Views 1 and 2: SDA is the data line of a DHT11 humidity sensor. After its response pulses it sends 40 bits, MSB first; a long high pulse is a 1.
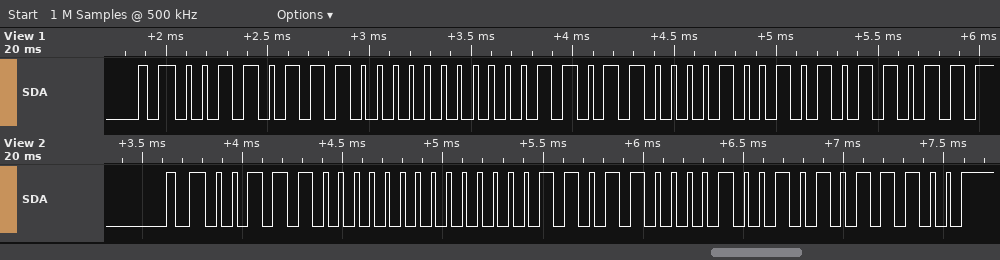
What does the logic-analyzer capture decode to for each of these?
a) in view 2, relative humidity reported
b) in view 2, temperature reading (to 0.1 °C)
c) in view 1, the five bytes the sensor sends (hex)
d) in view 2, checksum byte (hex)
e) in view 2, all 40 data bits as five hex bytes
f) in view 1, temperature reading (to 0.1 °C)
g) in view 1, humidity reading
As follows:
56 %
27.9 °C
37 00 1B 09 5B
0x5C
38 00 1B 09 5C
27.9 °C
55 %
